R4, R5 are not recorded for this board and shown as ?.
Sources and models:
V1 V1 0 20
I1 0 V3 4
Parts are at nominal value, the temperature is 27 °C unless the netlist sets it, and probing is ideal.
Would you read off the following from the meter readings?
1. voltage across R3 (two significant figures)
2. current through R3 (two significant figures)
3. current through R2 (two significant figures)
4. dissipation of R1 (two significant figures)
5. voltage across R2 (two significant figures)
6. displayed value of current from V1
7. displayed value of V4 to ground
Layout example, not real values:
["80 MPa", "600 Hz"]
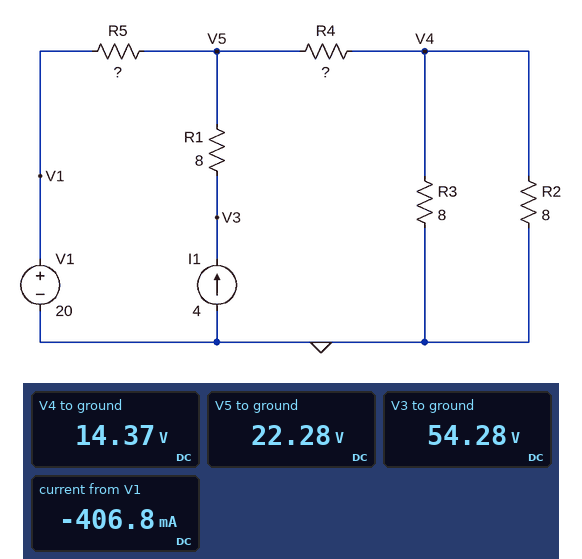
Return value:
["14 V", "1.8 A", "1.8 A", "130 W", "14 V", "-406.8 mA", "14.37 V"]
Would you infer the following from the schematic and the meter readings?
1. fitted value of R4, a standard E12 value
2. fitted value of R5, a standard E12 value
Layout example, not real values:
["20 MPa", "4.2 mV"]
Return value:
["2.2 Ω", "5.6 Ω"]
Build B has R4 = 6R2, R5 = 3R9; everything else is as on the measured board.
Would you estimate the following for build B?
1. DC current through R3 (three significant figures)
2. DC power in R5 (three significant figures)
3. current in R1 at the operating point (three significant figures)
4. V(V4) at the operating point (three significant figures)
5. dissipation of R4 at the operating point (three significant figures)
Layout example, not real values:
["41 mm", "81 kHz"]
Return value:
["1.26 A", "8.49 W", "4.00 A", "10.1 V", "39.5 W"]
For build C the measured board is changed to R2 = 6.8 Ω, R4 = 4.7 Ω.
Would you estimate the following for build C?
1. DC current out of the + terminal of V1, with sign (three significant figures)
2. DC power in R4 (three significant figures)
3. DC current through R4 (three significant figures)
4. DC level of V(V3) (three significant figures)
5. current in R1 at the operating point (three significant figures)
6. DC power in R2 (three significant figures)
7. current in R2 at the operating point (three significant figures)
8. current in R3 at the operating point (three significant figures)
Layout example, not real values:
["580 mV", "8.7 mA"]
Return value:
["-966 mA", "43.3 W", "3.03 A", "57.4 V", "4.00 A", "18.3 W", "1.64 A", "1.39 A"]
